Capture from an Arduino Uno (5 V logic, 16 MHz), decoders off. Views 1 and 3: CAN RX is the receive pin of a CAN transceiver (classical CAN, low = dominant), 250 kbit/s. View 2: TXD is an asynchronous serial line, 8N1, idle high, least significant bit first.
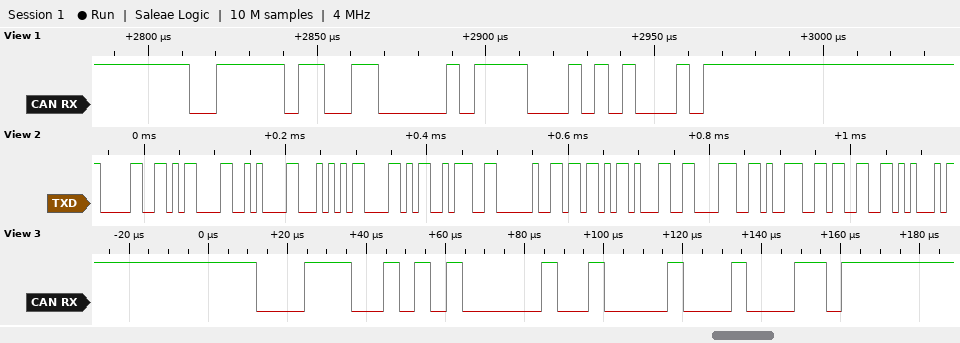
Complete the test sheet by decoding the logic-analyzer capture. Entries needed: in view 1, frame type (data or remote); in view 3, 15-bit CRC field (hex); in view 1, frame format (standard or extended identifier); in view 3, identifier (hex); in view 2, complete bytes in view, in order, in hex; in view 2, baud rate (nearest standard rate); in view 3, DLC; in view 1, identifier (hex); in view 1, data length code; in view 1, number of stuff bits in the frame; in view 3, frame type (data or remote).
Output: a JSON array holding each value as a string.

["remote", "0x2111", "standard", "0x1CA", "30 0D 0A 54 58 3A 20 5B 31 38 39 33 45", "115200 baud", "0", "0x3F9", "0", "2", "remote"]
